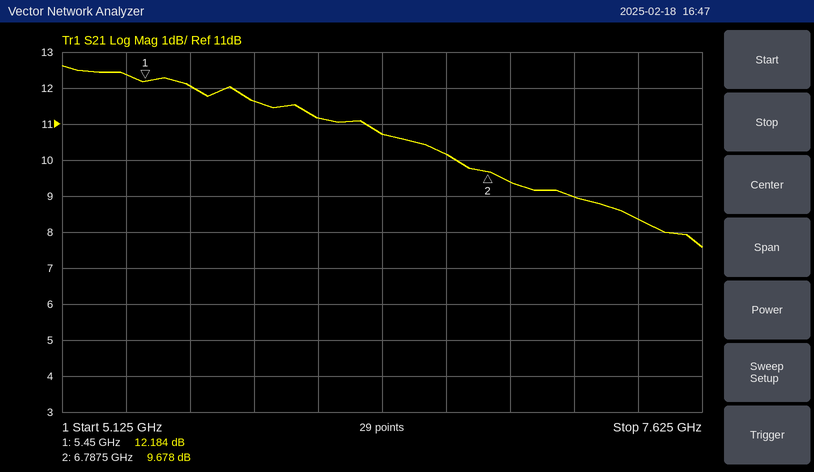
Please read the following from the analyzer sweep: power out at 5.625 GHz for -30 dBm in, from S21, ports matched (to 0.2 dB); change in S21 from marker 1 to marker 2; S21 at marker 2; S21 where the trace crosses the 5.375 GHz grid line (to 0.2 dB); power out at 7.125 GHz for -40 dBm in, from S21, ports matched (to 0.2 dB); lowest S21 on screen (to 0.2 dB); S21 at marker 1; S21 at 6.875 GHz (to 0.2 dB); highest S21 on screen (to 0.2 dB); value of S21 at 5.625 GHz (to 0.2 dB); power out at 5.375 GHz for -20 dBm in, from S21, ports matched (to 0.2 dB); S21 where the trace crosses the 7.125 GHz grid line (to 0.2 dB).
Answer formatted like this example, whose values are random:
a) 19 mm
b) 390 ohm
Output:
a) -18.0 dBm
b) -2.506 dB
c) 9.678 dB
d) 12.4 dB
e) -31.0 dBm
f) 7.6 dB
g) 12.184 dB
h) 9.4 dB
i) 12.6 dB
j) 12.0 dB
k) -7.6 dBm
l) 9.0 dB
